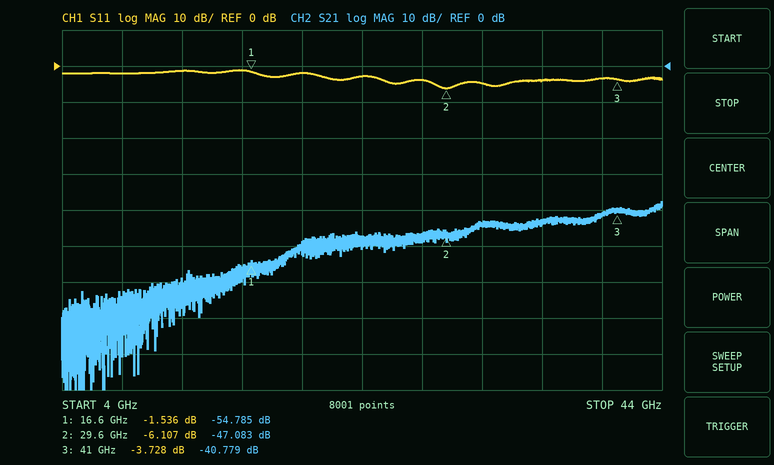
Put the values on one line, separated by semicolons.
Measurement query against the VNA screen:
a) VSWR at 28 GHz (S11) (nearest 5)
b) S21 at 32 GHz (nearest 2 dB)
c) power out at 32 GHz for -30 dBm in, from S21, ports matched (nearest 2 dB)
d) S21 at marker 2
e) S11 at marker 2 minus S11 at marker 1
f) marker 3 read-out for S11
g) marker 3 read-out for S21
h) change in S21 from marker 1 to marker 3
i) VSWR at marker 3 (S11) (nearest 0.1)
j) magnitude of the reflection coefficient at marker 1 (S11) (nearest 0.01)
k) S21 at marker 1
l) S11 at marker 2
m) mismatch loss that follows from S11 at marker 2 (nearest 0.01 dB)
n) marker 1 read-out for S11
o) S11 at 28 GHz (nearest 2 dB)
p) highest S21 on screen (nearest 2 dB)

5; -44 dB; -74 dBm; -47.083 dB; -4.571 dB; -3.728 dB; -40.779 dB; 14.006 dB; 4.7; 0.84; -54.785 dB; -6.107 dB; 1.22 dB; -1.536 dB; -4 dB; -38 dB
